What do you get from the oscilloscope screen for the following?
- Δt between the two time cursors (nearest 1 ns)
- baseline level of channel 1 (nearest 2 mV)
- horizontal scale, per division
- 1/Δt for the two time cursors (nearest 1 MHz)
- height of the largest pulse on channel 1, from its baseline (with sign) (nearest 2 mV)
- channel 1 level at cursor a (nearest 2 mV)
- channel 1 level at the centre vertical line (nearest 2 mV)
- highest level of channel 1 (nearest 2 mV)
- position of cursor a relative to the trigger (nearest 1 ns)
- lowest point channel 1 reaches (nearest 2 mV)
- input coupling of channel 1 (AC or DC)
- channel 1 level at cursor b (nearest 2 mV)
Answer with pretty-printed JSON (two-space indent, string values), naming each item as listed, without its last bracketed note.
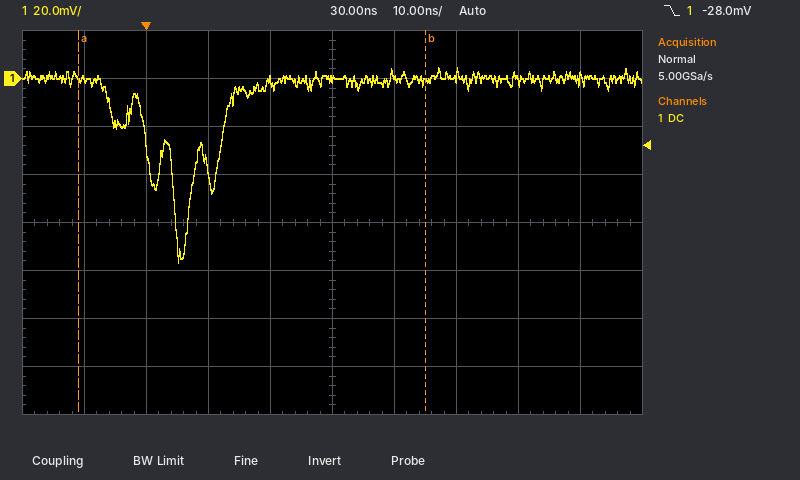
{
  "Δt between the two time cursors": "56 ns",
  "baseline level of channel 1": "0 mV",
  "horizontal scale, per division": "10 ns",
  "1/Δt for the two time cursors": "18 MHz",
  "height of the largest pulse on channel 1, from its baseline (with sign)": "-76 mV",
  "channel 1 level at cursor a": "0 mV",
  "channel 1 level at the centre vertical line": "0 mV",
  "highest level of channel 1": "4 mV",
  "position of cursor a relative to the trigger": "-11 ns",
  "lowest point channel 1 reaches": "-76 mV",
  "input coupling of channel 1": "DC",
  "channel 1 level at cursor b": "-2 mV"
}
